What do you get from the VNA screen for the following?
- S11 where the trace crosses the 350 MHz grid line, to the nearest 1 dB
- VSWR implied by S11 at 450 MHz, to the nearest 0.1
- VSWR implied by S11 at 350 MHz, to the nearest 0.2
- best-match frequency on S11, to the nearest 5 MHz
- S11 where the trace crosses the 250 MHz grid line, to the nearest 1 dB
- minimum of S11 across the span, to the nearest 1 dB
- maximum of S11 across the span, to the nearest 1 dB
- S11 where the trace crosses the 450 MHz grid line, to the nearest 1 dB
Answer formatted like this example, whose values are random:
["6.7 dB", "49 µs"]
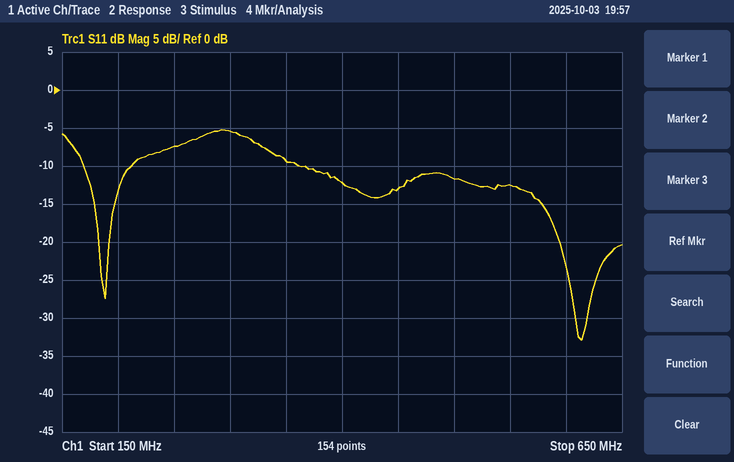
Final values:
["-9 dB", "1.6", "2.0", "615 MHz", "-7 dB", "-33 dB", "-5 dB", "-13 dB"]
